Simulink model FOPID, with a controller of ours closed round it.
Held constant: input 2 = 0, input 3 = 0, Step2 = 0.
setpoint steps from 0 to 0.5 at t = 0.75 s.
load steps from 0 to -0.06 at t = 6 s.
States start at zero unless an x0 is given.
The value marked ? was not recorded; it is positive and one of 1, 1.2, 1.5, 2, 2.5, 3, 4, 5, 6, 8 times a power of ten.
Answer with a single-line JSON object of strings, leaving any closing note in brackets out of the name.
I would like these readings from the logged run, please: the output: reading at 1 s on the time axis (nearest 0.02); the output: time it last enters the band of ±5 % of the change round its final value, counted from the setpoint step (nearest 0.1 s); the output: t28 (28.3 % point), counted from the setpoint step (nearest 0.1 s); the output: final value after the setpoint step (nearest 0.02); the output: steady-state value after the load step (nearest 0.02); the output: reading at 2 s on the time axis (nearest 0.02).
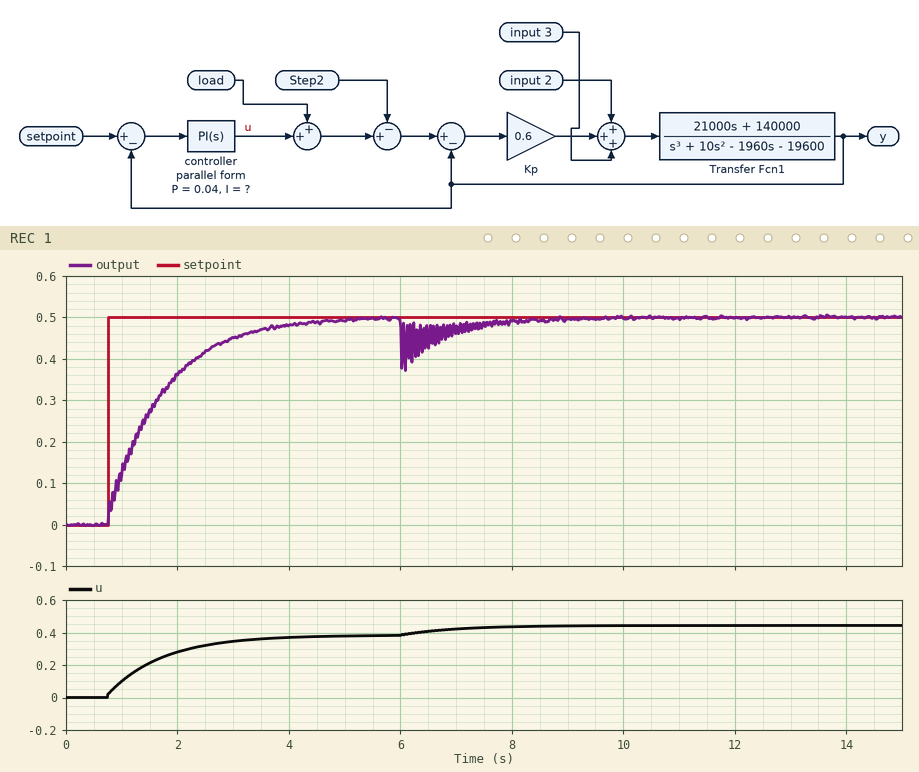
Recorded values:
{"the output: reading at 1 s on the time axis": "0.12", "the output: time it last enters the band of ±5 % of the change round its final value, counted from the setpoint step": "2.9 s", "the output: t28 (28.3 % point), counted from the setpoint step": "0.3 s", "the output: final value after the setpoint step": "0.50", "the output: steady-state value after the load step": "0.50", "the output: reading at 2 s on the time axis": "0.36"}
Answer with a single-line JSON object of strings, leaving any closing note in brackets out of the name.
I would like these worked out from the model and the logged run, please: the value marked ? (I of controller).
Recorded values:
{"the value marked ?": "0.8"}
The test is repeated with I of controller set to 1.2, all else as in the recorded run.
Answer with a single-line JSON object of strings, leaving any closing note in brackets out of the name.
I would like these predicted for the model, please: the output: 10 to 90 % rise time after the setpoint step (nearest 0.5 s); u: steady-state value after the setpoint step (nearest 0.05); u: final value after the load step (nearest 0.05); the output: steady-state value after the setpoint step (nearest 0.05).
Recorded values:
{"the output: 10 to 90 % rise time after the setpoint step": "1.5 s", "u: steady-state value after the setpoint step": "0.40", "u: final value after the load step": "0.45", "the output: steady-state value after the setpoint step": "0.50"}
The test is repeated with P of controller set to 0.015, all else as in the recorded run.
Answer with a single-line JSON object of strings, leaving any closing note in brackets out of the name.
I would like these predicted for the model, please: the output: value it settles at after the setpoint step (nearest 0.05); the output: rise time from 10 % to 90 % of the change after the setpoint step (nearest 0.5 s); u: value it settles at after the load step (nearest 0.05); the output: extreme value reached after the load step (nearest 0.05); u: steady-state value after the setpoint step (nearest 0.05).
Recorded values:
{"the output: value it settles at after the setpoint step": "0.50", "the output: rise time from 10 % to 90 % of the change after the setpoint step": "2.0 s", "u: value it settles at after the load step": "0.45", "the output: extreme value reached after the load step": "0.35", "u: steady-state value after the setpoint step": "0.40"}
